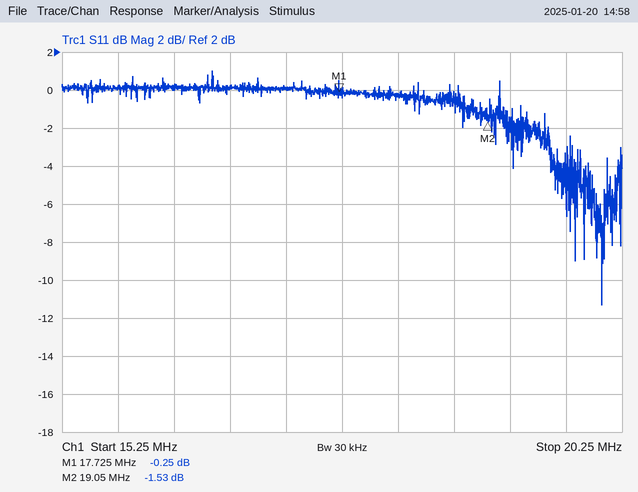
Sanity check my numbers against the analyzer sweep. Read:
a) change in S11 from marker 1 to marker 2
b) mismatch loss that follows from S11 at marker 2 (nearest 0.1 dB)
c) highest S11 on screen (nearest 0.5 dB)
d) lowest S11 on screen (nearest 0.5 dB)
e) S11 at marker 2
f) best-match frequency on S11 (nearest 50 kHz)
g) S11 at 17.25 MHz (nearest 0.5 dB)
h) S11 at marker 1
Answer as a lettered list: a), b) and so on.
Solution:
a) -1.28 dB
b) 5.3 dB
c) 1.0 dB
d) -11.5 dB
e) -1.53 dB
f) 20.05 MHz
g) 0.0 dB
h) -0.25 dB
